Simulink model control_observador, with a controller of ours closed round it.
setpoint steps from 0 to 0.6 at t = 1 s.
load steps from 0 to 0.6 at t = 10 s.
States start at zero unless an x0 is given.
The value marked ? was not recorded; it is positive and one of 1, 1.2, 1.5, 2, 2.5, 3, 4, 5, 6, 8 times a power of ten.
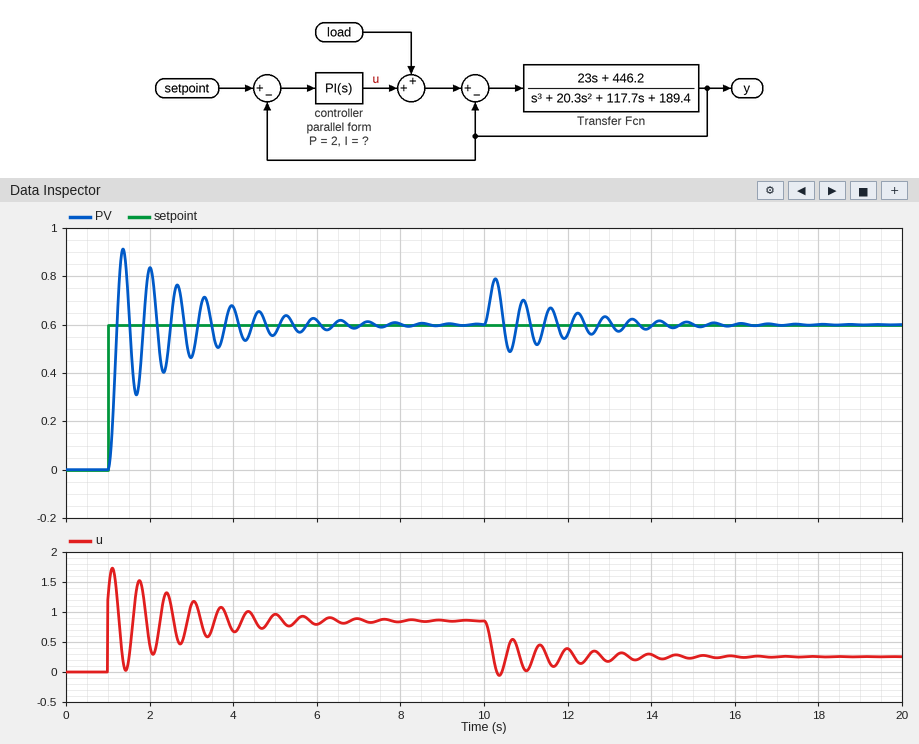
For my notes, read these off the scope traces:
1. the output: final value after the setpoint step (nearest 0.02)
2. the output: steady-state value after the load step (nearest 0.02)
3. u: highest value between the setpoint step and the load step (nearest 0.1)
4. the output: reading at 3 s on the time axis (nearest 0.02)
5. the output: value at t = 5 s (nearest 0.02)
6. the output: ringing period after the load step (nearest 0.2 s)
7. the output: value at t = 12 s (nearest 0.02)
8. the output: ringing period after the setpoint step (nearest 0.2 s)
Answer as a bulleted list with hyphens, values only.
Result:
- 0.60
- 0.60
- 1.7
- 0.46
- 0.56
- 0.6 s
- 0.56
- 0.6 s
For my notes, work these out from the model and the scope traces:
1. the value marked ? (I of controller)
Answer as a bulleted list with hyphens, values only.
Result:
- 15
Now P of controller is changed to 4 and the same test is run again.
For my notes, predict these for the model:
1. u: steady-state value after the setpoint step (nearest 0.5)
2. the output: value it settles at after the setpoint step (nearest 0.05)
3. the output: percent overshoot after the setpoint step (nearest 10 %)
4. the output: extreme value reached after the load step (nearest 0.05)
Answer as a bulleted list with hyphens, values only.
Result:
- 1.0
- 0.60
- 50 %
- 0.75
